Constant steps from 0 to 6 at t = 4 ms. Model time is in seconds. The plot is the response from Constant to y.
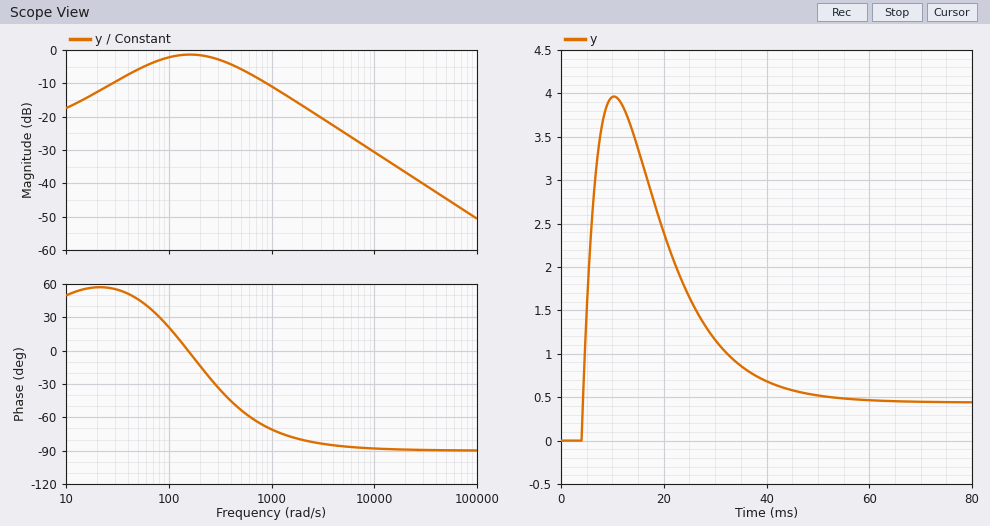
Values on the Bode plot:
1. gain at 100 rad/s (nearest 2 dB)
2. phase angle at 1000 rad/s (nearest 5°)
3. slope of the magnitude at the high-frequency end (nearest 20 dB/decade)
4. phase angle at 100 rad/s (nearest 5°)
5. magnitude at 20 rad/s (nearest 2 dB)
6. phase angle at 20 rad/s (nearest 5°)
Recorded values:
-2 dB
-70°
-20 dB/decade
20°
-12 dB
55°
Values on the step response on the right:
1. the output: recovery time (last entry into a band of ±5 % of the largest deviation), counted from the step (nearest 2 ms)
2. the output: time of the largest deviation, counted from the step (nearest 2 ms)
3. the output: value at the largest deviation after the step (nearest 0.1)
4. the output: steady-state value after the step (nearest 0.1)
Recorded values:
38 ms
6 ms
4.0
0.4
